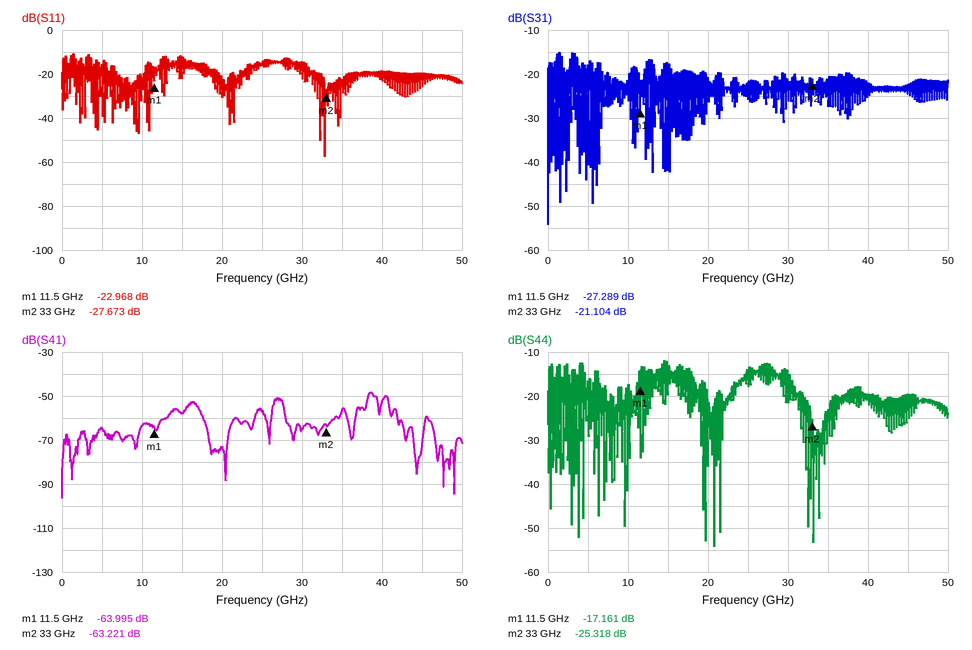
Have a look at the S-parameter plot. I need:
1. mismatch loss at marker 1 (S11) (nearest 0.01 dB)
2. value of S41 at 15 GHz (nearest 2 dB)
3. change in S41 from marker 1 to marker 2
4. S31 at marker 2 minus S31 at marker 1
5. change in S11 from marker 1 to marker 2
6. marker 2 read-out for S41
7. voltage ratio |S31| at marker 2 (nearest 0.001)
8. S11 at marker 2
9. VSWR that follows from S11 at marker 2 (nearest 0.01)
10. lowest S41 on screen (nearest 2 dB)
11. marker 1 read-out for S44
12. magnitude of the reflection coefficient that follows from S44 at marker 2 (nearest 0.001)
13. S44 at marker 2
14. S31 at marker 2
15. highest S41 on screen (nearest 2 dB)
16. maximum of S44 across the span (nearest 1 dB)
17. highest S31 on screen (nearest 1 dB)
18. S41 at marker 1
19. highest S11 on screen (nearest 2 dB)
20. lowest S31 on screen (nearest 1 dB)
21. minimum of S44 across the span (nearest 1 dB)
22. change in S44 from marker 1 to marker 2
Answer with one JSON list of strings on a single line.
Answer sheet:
["0.02 dB", "-58 dB", "0.774 dB", "6.185 dB", "-4.705 dB", "-63.221 dB", "0.088", "-27.673 dB", "1.09", "-96 dB", "-17.161 dB", "0.054", "-25.318 dB", "-21.104 dB", "-48 dB", "-12 dB", "-15 dB", "-63.995 dB", "-10 dB", "-54 dB", "-54 dB", "-8.157 dB"]
